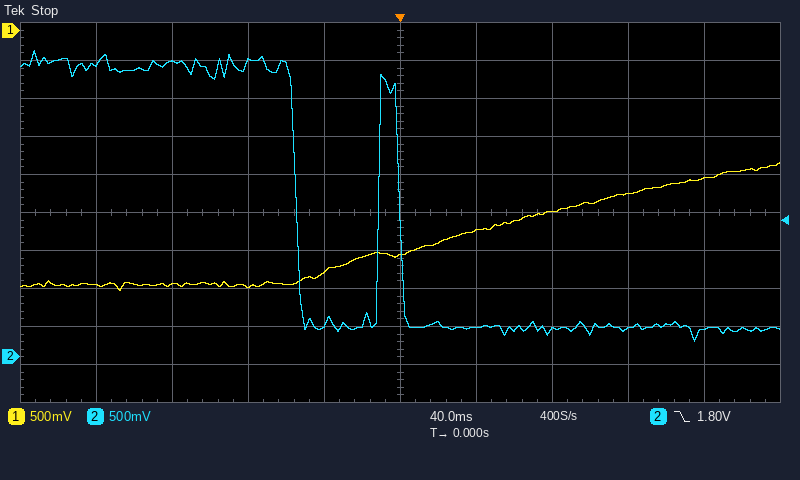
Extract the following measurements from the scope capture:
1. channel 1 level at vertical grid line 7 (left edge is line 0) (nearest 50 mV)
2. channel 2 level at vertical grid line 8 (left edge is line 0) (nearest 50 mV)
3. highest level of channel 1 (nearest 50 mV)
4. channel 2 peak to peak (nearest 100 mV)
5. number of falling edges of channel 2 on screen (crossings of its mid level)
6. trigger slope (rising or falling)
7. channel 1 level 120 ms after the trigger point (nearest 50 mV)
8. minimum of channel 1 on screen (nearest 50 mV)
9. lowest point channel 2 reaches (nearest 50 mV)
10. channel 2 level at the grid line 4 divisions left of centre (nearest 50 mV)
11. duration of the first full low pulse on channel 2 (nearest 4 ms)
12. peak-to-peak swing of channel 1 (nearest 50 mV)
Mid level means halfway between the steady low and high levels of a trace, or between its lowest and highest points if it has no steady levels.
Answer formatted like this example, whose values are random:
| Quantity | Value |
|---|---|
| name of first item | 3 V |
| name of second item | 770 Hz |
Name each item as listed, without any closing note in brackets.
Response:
| Quantity | Value |
|---|---|
| channel 1 level at vertical grid line 7 (left edge is line 0) | -2.40 V |
| channel 2 level at vertical grid line 8 (left edge is line 0) | 350 mV |
| highest level of channel 1 | -1.75 V |
| channel 2 peak to peak | 3.80 V |
| number of falling edges of channel 2 on screen | 2 |
| trigger slope | falling |
| channel 1 level 120 ms after the trigger point | -2.15 V |
| minimum of channel 1 on screen | -3.45 V |
| lowest point channel 2 reaches | 200 mV |
| channel 2 level at the grid line 4 divisions left of centre | 3.85 V |
| duration of the first full low pulse on channel 2 | 44 ms |
| peak-to-peak swing of channel 1 | 1.70 V |
